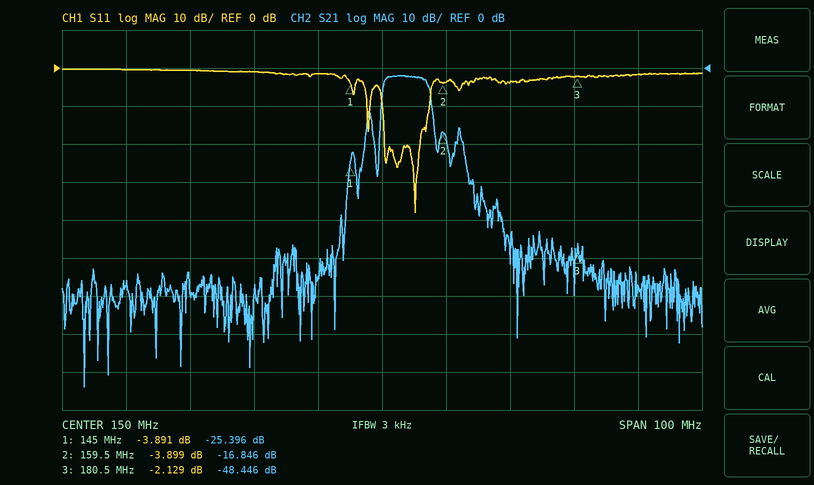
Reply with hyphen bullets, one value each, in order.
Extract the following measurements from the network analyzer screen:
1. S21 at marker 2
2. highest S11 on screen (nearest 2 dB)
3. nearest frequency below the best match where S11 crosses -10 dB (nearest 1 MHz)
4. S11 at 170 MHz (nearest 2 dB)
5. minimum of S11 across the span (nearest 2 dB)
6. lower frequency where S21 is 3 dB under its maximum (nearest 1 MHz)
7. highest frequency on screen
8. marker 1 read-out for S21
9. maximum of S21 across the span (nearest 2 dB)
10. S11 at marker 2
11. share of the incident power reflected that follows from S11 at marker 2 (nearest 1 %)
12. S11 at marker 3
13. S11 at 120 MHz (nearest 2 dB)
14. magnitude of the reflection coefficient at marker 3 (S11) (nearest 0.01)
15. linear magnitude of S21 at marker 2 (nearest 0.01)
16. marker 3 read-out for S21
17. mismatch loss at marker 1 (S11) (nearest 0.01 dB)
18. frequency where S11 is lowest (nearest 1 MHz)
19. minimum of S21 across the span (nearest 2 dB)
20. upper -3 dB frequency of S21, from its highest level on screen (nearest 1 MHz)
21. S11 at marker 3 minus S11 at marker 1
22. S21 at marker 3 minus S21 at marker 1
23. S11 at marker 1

- -16.846 dB
- 0 dB
- 150 MHz
- -4 dB
- -38 dB
- 150 MHz
- 200 MHz
- -25.396 dB
- -2 dB
- -3.899 dB
- 41 %
- -2.129 dB
- 0 dB
- 0.78
- 0.14
- -48.446 dB
- 2.28 dB
- 155 MHz
- -84 dB
- 157 MHz
- 1.762 dB
- -23.050 dB
- -3.891 dB
